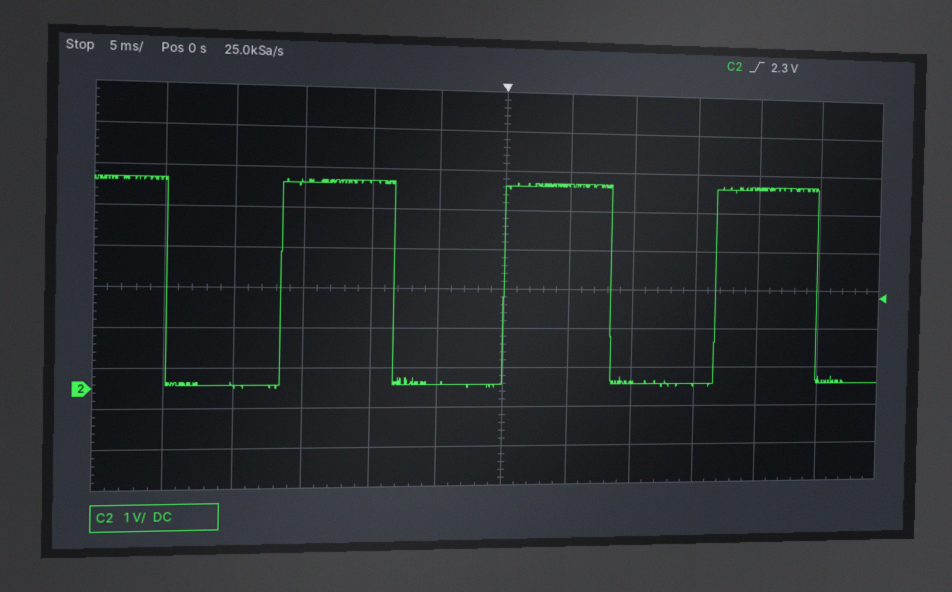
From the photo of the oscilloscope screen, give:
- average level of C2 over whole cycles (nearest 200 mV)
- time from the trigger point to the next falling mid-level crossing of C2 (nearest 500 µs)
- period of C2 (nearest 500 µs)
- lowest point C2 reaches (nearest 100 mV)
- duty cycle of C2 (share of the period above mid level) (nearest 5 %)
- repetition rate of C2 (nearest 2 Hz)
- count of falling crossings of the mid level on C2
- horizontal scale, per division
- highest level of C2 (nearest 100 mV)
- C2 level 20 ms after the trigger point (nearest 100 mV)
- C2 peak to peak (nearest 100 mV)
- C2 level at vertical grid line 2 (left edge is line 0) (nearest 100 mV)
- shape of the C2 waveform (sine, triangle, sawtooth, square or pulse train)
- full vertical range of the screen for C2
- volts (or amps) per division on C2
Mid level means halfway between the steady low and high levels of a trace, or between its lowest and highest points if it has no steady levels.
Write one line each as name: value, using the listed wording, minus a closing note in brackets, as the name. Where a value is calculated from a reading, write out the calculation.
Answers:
average level of C2 over whole cycles: 0.0 V + 0.5 × (5.2 V − (0.0 V)) ≈ 2.6 V
time from the trigger point to the next falling mid-level crossing of C2: 8.5 ms
period of C2: 16.5 ms
lowest point C2 reaches: 0.0 V
duty cycle of C2 (share of the period above mid level): 50 %
repetition rate of C2: 1 / 16.5 ms ≈ 60.6 Hz, so 60 Hz to the nearest 2 Hz
count of falling crossings of the mid level on C2: 4
horizontal scale, per division: 5 ms
highest level of C2: 5.2 V
C2 level 20 ms after the trigger point: 5.2 V
C2 peak to peak: 5.2 V − (0.0 V) = 5.2 V
C2 level at vertical grid line 2 (left edge is line 0): 100 mV
shape of the C2 waveform: square
full vertical range of the screen for C2: 10 V
volts (or amps) per division on C2: 1 V
